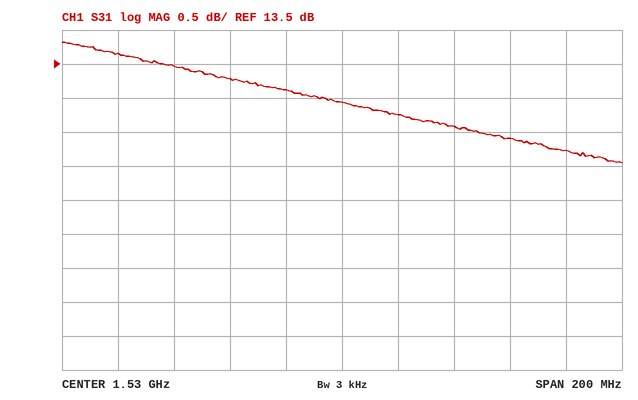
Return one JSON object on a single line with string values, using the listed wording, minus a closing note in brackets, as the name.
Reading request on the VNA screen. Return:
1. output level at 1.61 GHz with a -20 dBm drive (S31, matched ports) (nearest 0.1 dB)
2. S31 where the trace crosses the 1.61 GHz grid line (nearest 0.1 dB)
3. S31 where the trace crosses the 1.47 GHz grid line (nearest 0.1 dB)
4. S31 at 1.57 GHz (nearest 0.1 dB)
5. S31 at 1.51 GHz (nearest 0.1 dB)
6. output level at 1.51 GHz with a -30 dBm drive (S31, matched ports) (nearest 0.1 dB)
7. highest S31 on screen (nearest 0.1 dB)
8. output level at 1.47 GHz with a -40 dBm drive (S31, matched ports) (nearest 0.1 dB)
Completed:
{"output level at 1.61 GHz with a -20 dBm drive (S31, matched ports)": "-7.8 dBm", "S31 where the trace crosses the 1.61 GHz grid line": "12.2 dB", "S31 where the trace crosses the 1.47 GHz grid line": "13.5 dB", "S31 at 1.57 GHz": "12.6 dB", "S31 at 1.51 GHz": "13.1 dB", "output level at 1.51 GHz with a -30 dBm drive (S31, matched ports)": "-16.9 dBm", "highest S31 on screen": "13.8 dB", "output level at 1.47 GHz with a -40 dBm drive (S31, matched ports)": "-26.5 dBm"}
